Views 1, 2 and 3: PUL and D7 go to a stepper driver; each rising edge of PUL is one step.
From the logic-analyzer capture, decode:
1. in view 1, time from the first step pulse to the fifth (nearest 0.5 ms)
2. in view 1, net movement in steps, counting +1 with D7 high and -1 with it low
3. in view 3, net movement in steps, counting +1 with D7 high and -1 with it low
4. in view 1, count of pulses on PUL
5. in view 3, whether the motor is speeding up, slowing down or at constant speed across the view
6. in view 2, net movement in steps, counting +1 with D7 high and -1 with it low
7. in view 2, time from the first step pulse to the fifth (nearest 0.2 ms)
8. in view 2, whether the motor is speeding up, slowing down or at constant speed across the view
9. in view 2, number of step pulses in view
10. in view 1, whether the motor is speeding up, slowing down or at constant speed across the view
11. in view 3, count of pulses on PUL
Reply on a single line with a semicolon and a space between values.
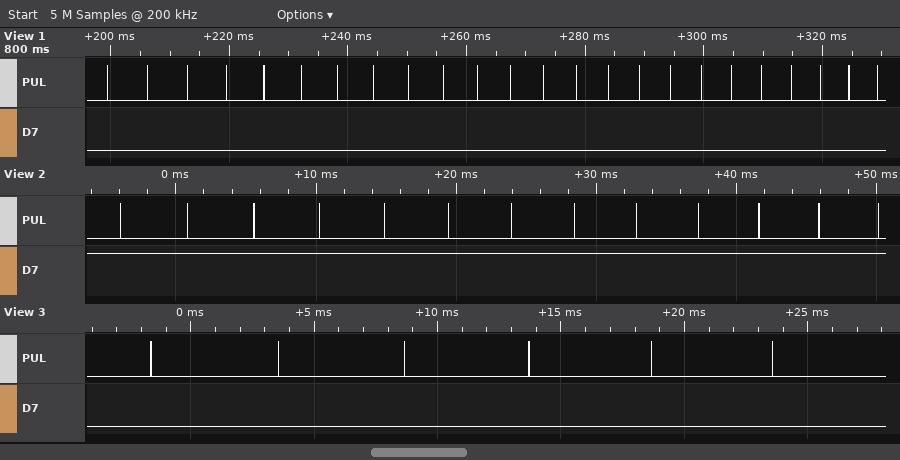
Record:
26.5 ms; -24; -6; 24; speeding up; +13; 18.8 ms; speeding up; 13; speeding up; 6
